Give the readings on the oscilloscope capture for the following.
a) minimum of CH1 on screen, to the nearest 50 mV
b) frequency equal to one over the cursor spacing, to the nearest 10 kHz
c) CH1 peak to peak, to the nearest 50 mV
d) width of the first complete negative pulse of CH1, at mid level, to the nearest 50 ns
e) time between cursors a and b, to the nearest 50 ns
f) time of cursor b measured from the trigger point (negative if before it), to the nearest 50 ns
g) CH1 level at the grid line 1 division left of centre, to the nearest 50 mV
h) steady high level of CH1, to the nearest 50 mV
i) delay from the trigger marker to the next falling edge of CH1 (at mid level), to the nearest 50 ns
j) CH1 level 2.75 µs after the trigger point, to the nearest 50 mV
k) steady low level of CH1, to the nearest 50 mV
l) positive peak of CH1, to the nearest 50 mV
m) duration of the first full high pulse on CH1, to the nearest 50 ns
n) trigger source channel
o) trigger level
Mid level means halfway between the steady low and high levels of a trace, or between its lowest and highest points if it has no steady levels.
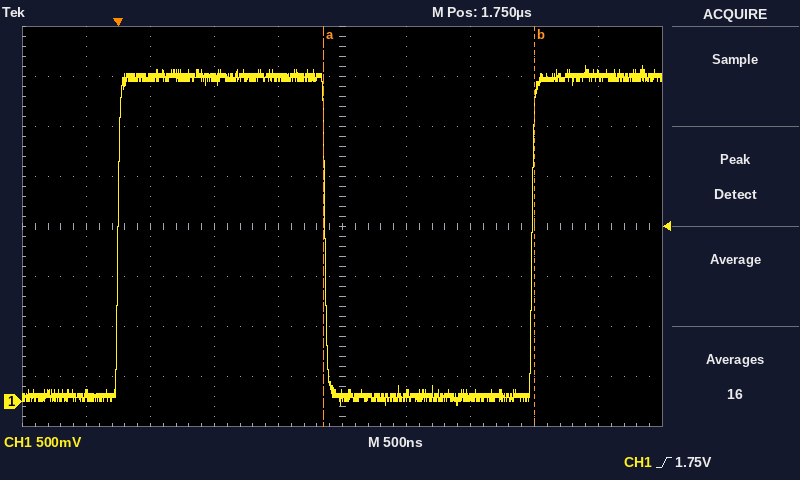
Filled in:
-50 mV
610 kHz
3.40 V
1.60 µs
1.65 µs
+3.25 µs
3.25 V
3.25 V
1.60 µs
50 mV
50 mV
3.35 V
1.60 µs
CH1
1.75 V
